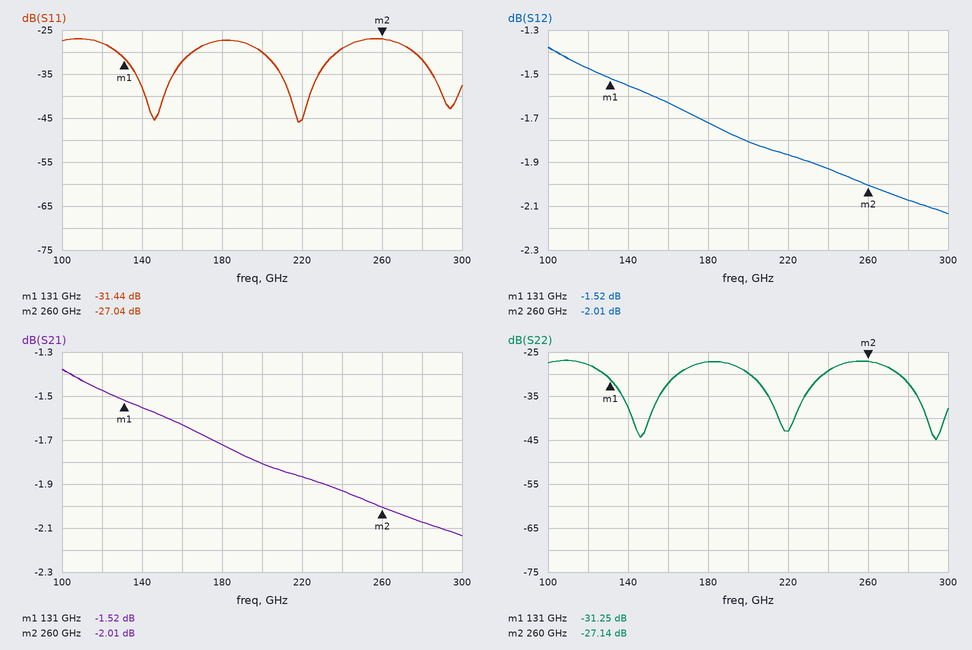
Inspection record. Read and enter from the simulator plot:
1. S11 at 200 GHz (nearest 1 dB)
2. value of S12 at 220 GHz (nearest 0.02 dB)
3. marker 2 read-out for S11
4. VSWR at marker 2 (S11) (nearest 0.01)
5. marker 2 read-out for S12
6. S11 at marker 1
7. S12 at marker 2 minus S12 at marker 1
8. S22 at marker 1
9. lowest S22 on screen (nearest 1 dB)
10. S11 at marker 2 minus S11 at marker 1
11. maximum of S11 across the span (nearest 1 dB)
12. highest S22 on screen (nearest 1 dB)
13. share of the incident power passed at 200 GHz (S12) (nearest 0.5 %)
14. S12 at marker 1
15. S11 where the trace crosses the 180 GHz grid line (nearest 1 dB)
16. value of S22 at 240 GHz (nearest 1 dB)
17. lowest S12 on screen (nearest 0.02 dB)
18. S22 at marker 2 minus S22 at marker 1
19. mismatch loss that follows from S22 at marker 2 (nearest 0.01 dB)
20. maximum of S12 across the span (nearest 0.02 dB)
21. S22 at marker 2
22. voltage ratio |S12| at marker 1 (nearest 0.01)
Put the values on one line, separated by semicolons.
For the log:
-30 dB; -1.86 dB; -27.04 dB; 1.09; -2.01 dB; -31.44 dB; -0.49 dB; -31.25 dB; -45 dB; 4.40 dB; -27 dB; -27 dB; 66.0 %; -1.52 dB; -27 dB; -29 dB; -2.14 dB; 4.11 dB; 0.01 dB; -1.38 dB; -27.14 dB; 0.84
